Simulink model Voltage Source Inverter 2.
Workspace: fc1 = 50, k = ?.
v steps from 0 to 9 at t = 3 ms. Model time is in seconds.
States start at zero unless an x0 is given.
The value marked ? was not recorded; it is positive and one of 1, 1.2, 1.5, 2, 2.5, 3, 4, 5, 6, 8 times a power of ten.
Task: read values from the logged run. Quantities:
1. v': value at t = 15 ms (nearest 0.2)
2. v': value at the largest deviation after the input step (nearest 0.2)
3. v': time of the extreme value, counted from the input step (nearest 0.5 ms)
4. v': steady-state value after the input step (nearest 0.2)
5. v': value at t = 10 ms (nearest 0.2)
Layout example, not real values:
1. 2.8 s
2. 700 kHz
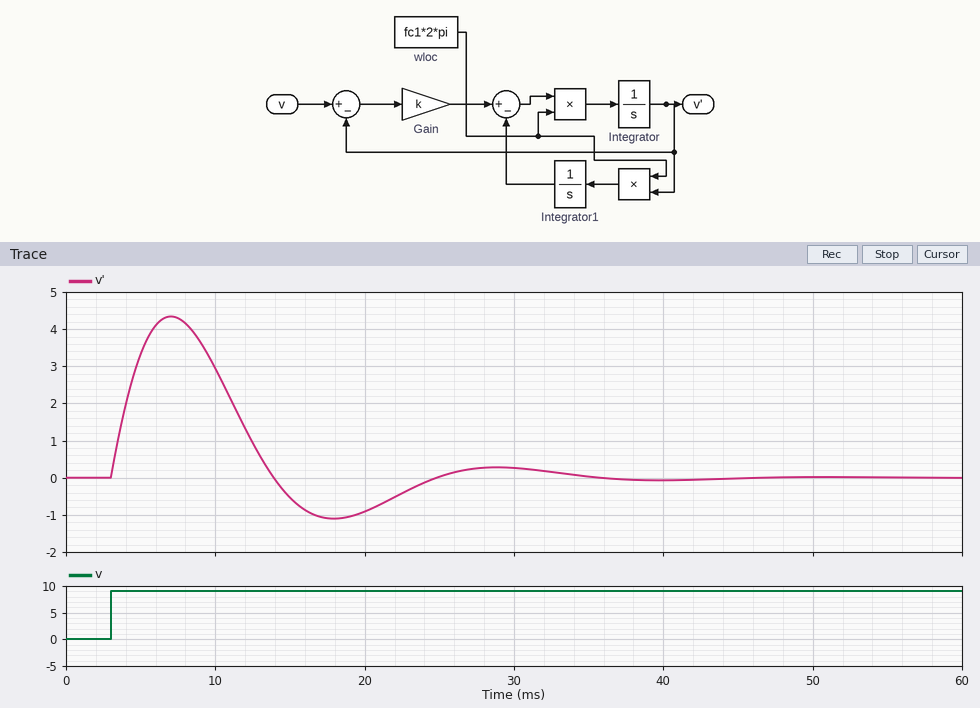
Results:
1. -0.6
2. 4.4
3. 4.0 ms
4. 0.0
5. 3.0
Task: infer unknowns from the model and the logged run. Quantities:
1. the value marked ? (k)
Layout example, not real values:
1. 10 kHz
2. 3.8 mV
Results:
1. 0.8
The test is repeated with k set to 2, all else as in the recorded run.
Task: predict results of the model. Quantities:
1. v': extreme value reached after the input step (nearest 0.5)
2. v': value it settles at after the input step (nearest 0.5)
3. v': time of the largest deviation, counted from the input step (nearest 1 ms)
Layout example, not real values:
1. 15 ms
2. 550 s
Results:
1. 6.5
2. 0.0
3. 3 ms
